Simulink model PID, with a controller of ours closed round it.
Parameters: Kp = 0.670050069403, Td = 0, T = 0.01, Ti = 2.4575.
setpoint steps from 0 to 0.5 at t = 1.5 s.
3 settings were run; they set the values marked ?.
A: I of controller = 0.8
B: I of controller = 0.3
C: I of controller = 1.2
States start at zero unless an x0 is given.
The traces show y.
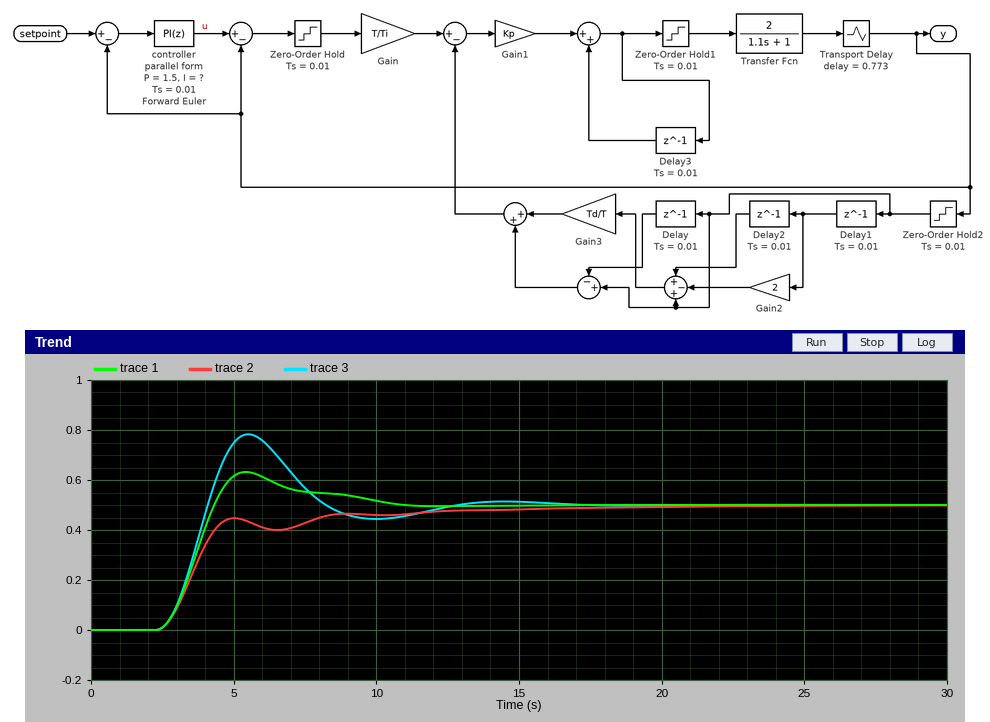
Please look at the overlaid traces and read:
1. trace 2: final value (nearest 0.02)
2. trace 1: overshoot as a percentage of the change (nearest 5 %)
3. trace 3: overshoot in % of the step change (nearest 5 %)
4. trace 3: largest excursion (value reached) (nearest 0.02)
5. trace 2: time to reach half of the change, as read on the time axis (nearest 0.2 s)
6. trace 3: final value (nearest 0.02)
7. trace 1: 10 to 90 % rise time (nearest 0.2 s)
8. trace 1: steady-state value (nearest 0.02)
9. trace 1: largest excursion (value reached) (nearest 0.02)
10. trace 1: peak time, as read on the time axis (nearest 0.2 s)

0.50
25 %
55 %
0.78
3.6 s
0.50
1.4 s
0.50
0.64
5.4 s
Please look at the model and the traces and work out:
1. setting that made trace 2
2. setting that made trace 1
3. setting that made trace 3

B
A
C
